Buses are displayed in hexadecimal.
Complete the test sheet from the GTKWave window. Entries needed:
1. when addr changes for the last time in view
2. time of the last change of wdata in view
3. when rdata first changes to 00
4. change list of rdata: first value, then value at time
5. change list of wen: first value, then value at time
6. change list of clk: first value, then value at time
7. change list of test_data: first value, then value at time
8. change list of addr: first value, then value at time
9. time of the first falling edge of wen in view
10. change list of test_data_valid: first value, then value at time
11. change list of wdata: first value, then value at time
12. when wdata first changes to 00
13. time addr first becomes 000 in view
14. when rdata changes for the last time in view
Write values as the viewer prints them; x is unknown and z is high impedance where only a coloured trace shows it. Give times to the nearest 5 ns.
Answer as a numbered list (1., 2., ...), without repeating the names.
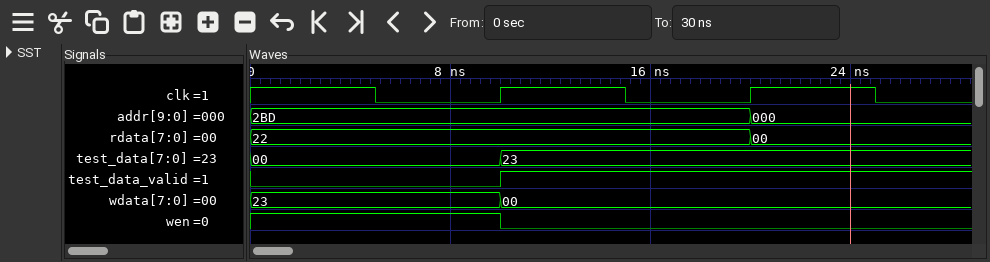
1. 20 ns
2. 10 ns
3. 20 ns
4. 22, 00 at 20 ns
5. 1, 0 at 10 ns
6. 1, 0 at 5 ns, 1 at 10 ns, 0 at 15 ns, 1 at 20 ns, 0 at 25 ns
7. 00, 23 at 10 ns
8. 2BD, 000 at 20 ns
9. 10 ns
10. 0, 1 at 10 ns
11. 23, 00 at 10 ns
12. 10 ns
13. 20 ns
14. 20 ns
